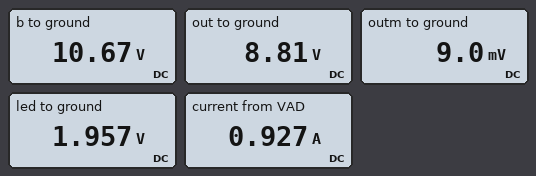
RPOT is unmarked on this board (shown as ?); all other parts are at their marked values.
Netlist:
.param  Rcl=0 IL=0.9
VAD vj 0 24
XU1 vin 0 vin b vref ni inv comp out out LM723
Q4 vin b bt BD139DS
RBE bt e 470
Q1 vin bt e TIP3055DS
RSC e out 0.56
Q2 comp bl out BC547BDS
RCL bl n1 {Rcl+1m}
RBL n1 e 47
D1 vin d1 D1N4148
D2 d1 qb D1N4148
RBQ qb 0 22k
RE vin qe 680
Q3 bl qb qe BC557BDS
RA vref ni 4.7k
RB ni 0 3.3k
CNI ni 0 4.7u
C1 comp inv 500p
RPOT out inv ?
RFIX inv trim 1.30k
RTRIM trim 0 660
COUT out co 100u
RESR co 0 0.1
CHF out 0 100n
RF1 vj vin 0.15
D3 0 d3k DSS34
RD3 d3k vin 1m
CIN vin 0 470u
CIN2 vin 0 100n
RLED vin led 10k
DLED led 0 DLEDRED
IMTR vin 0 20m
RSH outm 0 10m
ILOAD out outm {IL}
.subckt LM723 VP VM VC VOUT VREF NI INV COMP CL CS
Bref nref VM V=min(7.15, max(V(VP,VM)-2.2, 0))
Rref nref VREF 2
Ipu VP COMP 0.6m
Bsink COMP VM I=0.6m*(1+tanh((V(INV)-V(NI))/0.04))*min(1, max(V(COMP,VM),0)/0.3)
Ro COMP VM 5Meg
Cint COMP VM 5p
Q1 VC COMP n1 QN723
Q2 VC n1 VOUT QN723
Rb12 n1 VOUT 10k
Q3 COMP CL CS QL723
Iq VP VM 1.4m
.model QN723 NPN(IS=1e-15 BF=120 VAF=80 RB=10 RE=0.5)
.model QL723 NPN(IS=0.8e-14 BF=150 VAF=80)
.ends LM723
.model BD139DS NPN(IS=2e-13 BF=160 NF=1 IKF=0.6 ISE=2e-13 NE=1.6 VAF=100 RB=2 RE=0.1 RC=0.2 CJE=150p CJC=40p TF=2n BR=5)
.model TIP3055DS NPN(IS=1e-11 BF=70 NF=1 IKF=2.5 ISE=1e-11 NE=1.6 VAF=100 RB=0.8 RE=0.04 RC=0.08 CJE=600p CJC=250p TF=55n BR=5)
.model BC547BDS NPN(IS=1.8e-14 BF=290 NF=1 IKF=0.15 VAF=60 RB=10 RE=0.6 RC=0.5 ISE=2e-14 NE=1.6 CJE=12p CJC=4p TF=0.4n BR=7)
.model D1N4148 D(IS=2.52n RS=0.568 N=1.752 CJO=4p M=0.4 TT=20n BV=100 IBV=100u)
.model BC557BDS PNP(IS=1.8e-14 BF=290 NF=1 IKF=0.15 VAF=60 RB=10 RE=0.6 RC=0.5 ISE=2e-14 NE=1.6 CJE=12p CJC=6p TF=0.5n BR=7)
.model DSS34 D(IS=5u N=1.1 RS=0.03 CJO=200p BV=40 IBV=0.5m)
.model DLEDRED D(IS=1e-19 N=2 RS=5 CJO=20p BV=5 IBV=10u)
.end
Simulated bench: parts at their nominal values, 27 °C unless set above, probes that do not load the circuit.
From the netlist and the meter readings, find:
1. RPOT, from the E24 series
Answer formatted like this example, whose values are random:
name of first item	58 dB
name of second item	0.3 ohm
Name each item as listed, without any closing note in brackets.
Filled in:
RPOT, from the E24 series	3.9 kΩ
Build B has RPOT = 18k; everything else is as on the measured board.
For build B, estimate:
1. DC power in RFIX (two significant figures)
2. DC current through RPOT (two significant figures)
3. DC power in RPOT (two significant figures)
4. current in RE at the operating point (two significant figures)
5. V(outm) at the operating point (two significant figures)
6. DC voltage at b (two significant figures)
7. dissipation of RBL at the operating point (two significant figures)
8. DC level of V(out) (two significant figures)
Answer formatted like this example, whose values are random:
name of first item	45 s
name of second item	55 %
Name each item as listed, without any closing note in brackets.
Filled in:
DC power in RFIX	1.5 mW
DC current through RPOT	1.1 mA
DC power in RPOT	21 mW
current in RE at the operating point	790 µA
V(outm) at the operating point	9.0 mV
DC voltage at b	23 V
dissipation of RBL at the operating point	29 µW
DC level of V(out)	21 V
